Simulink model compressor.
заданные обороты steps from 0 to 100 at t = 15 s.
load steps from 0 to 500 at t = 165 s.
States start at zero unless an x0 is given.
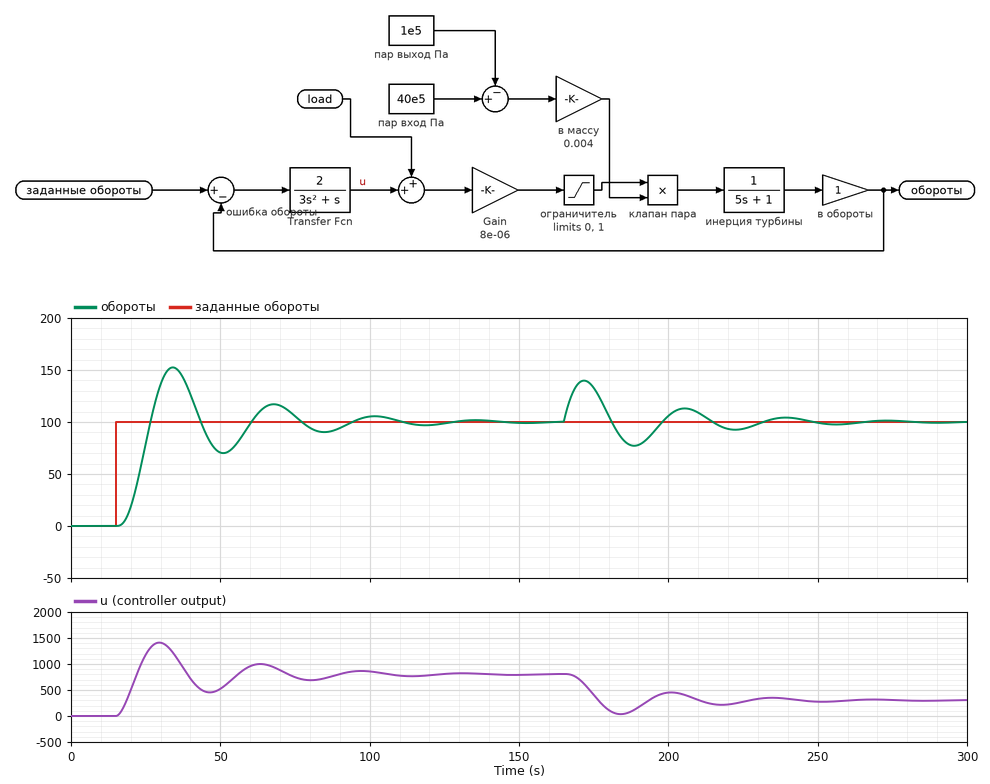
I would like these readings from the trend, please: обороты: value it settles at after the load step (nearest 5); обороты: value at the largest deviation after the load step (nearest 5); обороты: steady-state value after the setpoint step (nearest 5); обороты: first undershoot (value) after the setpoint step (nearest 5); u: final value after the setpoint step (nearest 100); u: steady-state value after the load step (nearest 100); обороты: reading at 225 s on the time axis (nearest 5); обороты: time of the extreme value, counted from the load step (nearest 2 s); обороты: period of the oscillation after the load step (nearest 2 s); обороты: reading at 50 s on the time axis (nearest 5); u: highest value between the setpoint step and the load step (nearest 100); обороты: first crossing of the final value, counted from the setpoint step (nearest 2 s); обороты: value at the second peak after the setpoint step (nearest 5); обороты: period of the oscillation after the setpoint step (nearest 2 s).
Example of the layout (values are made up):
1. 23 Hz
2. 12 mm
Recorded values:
1. 100
2. 140
3. 100
4. 70
5. 800
6. 300
7. 95
8. 6 s
9. 34 s
10. 70
11. 1400
12. 12 s
13. 115
14. 34 s
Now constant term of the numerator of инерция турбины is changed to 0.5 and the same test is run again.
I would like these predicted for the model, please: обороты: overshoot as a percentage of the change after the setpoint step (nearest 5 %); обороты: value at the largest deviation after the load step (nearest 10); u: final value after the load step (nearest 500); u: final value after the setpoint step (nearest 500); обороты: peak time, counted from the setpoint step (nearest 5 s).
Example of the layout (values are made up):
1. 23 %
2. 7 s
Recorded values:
1. 25 %
2. 120
3. 1000
4. 1500
5. 25 s
